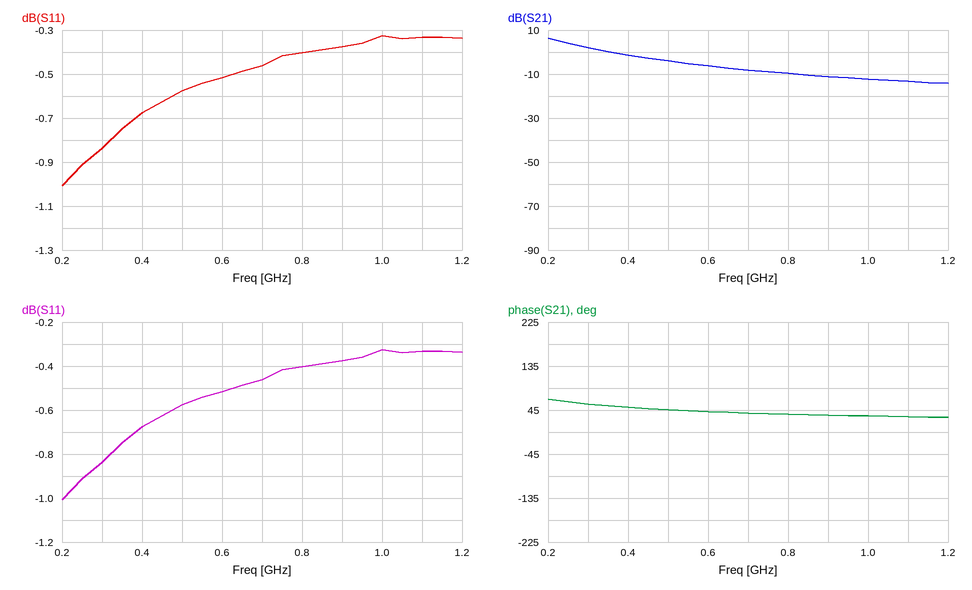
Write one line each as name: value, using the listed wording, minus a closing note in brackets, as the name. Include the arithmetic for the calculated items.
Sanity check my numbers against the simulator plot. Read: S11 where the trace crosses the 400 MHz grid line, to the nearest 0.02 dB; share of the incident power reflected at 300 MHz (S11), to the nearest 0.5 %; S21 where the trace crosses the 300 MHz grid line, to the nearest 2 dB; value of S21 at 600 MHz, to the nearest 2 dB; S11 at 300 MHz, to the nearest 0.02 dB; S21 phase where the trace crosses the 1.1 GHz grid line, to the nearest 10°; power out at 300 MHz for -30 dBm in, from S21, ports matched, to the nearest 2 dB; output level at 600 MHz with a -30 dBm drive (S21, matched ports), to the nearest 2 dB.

S11 where the trace crosses the 400 MHz grid line, to the nearest 0.02 dB: -0.68 dB
share of the incident power reflected at 300 MHz (S11), to the nearest 0.5 %: 10^(-0.84/10) ≈ 82.4 %, so 82.5 % to the nearest 0.5 %
S21 where the trace crosses the 300 MHz grid line, to the nearest 2 dB: 2 dB
value of S21 at 600 MHz, to the nearest 2 dB: -6 dB
S11 at 300 MHz, to the nearest 0.02 dB: -0.84 dB
S21 phase where the trace crosses the 1.1 GHz grid line, to the nearest 10°: 30°
power out at 300 MHz for -30 dBm in, from S21, ports matched, to the nearest 2 dB: -30 dBm + (2 dB) = -28 dBm
output level at 600 MHz with a -30 dBm drive (S21, matched ports), to the nearest 2 dB: -30 dBm + (-6 dB) = -36 dBm
